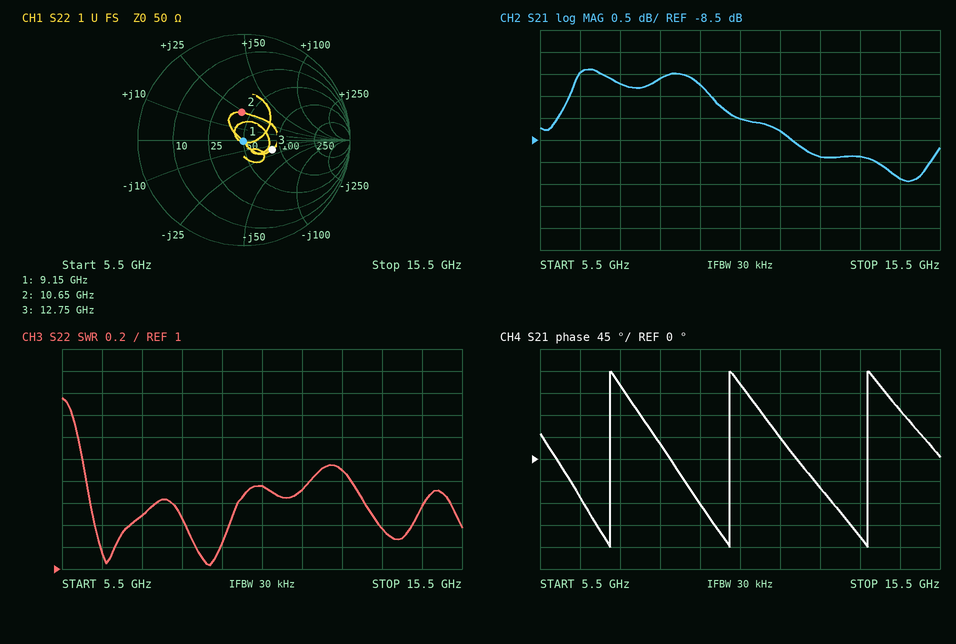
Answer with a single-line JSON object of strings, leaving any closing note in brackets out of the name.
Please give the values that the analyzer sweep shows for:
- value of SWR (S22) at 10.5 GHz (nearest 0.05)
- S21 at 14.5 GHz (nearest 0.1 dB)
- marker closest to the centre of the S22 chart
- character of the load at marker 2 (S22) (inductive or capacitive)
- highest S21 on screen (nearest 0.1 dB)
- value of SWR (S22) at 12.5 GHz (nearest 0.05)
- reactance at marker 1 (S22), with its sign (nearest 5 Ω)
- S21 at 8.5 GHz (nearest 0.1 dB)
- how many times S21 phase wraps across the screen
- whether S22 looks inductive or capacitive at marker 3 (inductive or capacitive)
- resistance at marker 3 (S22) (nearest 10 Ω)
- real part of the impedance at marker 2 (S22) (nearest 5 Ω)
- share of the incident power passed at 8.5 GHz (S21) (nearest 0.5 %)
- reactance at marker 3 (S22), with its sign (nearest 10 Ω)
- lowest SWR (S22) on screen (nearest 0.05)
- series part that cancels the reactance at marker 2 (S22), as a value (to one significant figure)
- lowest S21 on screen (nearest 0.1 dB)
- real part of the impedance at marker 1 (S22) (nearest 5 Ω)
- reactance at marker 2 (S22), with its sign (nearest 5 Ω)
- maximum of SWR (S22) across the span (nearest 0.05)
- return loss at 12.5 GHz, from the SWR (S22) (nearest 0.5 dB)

{"value of SWR (S22) at 10.5 GHz": "1.75", "S21 at 14.5 GHz": "-9.4 dB", "marker closest to the centre of the S22 chart": "marker 1", "character of the load at marker 2 (S22)": "inductive", "highest S21 on screen": "-6.9 dB", "value of SWR (S22) at 12.5 GHz": "1.90", "reactance at marker 1 (S22), with its sign": "0 Ω", "S21 at 8.5 GHz": "-7.1 dB", "how many times S21 phase wraps across the screen": "3", "whether S22 looks inductive or capacitive at marker 3": "capacitive", "resistance at marker 3 (S22)": "80 Ω", "real part of the impedance at marker 2 (S22)": "40 Ω", "share of the incident power passed at 8.5 GHz (S21)": "19.5 %", "reactance at marker 3 (S22), with its sign": "-20 Ω", "lowest SWR (S22) on screen": "1.05", "series part that cancels the reactance at marker 2 (S22), as a value": "600 fF", "lowest S21 on screen": "-9.4 dB", "real part of the impedance at marker 1 (S22)": "50 Ω", "reactance at marker 2 (S22), with its sign": "+25 Ω", "maximum of SWR (S22) across the span": "2.55", "return loss at 12.5 GHz, from the SWR (S22)": "10.0 dB"}
